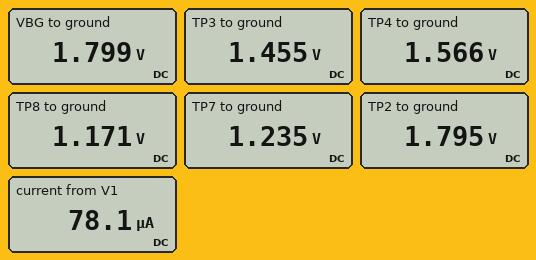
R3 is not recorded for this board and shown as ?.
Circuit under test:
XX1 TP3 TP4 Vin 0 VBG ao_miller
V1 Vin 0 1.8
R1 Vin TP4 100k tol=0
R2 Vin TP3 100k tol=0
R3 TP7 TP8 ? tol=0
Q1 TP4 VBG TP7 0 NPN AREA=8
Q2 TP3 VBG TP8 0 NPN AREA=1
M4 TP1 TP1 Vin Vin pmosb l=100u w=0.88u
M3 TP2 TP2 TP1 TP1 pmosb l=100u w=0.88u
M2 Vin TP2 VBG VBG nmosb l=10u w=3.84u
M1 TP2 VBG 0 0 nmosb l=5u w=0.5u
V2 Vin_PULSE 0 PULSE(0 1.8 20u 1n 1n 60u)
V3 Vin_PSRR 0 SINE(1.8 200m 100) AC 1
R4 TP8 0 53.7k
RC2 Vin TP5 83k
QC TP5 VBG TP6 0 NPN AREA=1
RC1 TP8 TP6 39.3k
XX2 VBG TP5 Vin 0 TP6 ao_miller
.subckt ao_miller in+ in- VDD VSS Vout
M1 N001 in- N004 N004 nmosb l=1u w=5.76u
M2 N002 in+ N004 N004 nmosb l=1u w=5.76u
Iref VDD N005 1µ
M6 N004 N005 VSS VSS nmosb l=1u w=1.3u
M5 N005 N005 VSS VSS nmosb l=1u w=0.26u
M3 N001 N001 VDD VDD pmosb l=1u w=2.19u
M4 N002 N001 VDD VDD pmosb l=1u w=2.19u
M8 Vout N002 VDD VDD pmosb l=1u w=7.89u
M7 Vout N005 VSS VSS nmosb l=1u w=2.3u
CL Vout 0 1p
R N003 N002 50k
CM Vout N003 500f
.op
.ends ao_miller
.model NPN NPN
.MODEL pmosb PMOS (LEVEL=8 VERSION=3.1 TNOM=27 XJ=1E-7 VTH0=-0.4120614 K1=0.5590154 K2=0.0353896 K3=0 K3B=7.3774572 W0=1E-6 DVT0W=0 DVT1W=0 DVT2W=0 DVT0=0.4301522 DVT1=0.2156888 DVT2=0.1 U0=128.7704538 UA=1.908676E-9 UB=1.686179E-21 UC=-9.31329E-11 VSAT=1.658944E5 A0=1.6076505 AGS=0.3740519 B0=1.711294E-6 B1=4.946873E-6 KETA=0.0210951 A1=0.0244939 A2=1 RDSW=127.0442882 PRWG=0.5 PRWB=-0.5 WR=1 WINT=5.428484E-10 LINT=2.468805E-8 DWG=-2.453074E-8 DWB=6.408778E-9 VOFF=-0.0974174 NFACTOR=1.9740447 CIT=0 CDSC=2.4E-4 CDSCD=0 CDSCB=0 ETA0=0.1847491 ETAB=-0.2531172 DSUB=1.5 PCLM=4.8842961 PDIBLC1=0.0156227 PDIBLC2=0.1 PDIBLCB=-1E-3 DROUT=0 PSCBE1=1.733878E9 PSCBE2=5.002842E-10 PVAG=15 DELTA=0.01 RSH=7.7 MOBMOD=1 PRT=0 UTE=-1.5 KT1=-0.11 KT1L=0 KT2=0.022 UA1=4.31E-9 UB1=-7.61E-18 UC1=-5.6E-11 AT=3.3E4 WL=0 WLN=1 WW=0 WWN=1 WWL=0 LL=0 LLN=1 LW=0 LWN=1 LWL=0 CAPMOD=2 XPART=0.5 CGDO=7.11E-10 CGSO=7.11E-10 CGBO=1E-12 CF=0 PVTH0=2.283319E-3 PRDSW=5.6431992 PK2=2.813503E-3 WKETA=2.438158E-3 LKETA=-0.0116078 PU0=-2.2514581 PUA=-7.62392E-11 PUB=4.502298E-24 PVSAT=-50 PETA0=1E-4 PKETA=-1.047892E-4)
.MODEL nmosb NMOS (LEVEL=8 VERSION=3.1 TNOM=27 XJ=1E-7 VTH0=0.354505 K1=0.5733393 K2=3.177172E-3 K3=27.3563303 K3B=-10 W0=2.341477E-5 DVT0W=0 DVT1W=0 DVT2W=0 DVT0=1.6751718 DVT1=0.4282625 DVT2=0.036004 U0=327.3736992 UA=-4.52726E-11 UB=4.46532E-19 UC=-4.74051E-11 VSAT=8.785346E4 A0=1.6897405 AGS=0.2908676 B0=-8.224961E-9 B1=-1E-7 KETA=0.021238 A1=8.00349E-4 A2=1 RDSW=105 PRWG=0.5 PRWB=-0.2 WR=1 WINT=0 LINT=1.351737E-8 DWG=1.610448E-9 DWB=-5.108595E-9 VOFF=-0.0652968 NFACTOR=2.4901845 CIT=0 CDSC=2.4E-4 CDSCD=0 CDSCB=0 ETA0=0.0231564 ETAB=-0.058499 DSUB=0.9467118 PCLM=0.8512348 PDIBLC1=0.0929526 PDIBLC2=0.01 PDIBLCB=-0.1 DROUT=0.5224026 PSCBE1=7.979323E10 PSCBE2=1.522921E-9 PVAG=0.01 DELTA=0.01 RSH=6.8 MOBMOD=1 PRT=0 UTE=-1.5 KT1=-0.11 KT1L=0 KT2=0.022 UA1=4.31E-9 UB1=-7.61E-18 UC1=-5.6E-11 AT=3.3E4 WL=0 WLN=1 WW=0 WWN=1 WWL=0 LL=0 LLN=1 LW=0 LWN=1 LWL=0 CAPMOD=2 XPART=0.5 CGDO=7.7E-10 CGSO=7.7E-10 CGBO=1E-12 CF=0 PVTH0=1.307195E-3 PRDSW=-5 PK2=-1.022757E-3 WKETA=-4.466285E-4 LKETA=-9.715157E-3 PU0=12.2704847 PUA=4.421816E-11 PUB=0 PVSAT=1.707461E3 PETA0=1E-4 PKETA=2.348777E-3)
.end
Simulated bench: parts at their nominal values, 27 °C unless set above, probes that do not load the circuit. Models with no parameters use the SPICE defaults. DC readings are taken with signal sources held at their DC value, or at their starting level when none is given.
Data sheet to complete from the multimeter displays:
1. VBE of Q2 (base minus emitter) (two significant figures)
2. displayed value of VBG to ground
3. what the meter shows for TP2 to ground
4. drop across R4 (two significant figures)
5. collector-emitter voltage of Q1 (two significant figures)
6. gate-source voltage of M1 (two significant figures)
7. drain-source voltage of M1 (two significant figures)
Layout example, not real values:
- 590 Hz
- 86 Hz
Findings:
- 630 mV
- 1.799 V
- 1.795 V
- 1.2 V
- 330 mV
- 1.8 V
- 1.8 V
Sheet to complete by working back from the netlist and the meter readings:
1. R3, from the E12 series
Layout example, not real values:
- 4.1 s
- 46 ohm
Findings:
- 27 kΩ
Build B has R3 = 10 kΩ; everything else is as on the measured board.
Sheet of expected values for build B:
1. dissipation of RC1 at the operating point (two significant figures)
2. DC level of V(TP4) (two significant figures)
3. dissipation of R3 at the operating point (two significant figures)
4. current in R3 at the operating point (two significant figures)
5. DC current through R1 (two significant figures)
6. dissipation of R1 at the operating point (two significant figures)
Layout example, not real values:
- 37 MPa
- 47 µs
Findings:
- 9.7 µW
- 1.4 V
- 160 nW
- 4.0 µA
- 3.9 µA
- 1.5 µW
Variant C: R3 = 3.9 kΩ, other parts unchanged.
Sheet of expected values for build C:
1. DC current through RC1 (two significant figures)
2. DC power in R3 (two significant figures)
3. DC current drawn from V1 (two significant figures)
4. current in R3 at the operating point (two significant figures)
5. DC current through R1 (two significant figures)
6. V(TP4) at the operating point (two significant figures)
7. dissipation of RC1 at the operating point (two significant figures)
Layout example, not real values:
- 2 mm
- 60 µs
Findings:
- 15 µA
- 110 nW
- 79 µA
- 5.2 µA
- 4.7 µA
- 1.3 V
- 9.4 µW
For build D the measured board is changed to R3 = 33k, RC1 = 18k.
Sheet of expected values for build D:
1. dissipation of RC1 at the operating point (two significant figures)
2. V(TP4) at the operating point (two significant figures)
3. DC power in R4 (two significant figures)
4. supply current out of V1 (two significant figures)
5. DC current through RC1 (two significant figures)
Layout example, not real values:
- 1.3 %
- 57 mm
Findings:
- 11 µW
- 1.8 V
- 34 µW
- 82 µA
- 25 µA
